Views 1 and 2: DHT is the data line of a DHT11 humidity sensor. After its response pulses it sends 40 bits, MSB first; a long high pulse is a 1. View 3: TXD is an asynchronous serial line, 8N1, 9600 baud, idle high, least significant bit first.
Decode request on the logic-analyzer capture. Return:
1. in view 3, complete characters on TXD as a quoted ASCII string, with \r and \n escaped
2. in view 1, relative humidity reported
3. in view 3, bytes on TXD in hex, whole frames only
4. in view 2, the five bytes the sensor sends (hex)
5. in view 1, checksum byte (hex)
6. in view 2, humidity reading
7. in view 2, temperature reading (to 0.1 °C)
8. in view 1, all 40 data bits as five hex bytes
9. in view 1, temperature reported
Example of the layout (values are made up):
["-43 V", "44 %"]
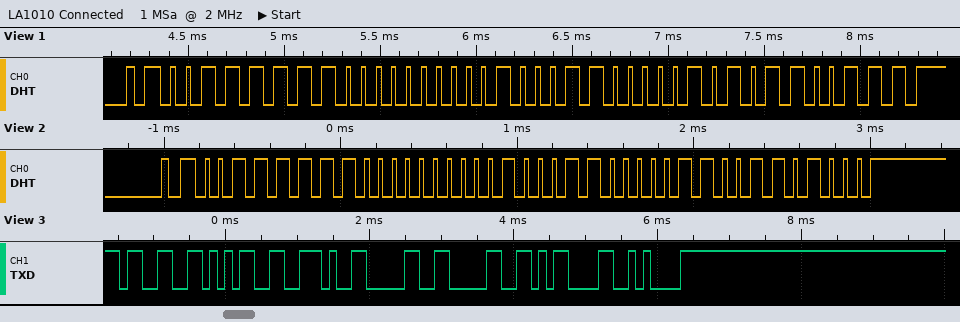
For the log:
["\"35.00\\r\\n\"", "63 %", "0x33 0x35 0x2E 0x30 0x30 0x0D 0x0A", "3F 00 23 06 68", "0x67", "63 %", "35.6 °C", "3F 00 23 05 67", "35.5 °C"]
